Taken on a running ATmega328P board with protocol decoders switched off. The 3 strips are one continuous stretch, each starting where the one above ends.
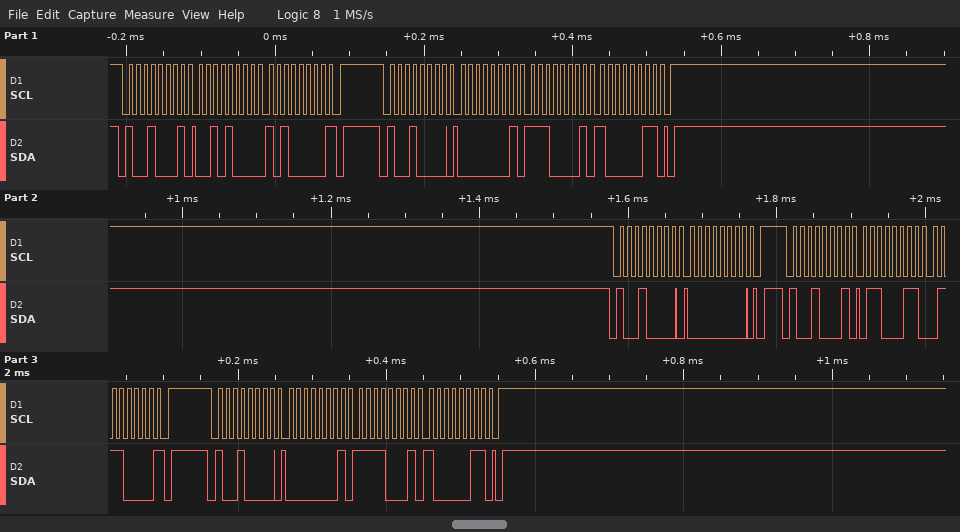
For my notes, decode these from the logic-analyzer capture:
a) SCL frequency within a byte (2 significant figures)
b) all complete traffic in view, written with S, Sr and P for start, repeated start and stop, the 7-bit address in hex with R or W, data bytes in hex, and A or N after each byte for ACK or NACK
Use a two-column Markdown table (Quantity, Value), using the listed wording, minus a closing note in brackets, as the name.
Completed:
| Quantity | Value |
|---|---|
| SCL frequency within a byte | 100 kHz |
| all complete traffic in view, written with S, Sr and P for start, repeated start and stop, the 7-bit address in hex with R or W, data bytes in hex, and A or N after each byte for ACK or NACK | S 48R A 28 A A0 N P S 48W A 01 A E1 A 83 A P S 48W A 00 A P S 48R A 63 A 70 N P S 48W A 01 A F1 A 83 A P |
